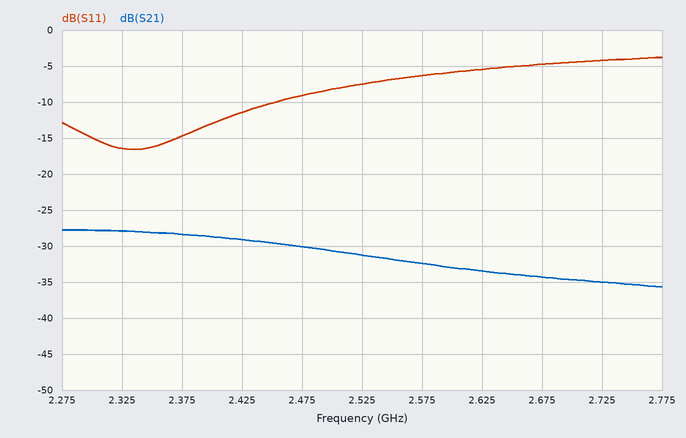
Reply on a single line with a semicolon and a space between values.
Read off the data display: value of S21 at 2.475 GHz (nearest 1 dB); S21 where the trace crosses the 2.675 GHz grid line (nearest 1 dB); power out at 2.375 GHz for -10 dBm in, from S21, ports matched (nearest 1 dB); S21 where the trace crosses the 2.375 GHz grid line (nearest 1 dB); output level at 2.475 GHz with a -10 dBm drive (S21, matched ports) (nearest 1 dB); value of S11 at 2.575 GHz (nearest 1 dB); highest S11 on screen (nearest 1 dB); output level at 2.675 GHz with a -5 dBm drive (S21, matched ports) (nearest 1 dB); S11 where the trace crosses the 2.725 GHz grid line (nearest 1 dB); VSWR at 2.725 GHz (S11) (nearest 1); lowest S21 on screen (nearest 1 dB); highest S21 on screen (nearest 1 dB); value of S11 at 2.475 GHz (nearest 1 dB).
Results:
-30 dB; -34 dB; -38 dBm; -28 dB; -40 dBm; -6 dB; -4 dB; -39 dBm; -4 dB; 4; -36 dB; -28 dB; -9 dB
